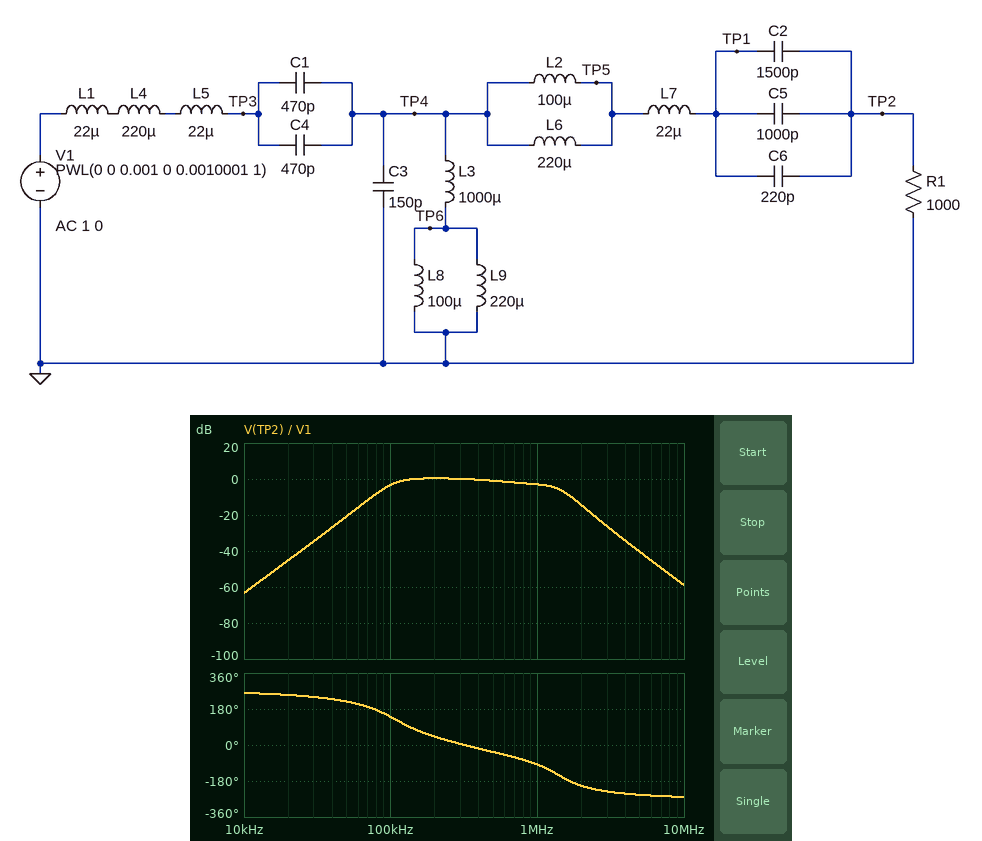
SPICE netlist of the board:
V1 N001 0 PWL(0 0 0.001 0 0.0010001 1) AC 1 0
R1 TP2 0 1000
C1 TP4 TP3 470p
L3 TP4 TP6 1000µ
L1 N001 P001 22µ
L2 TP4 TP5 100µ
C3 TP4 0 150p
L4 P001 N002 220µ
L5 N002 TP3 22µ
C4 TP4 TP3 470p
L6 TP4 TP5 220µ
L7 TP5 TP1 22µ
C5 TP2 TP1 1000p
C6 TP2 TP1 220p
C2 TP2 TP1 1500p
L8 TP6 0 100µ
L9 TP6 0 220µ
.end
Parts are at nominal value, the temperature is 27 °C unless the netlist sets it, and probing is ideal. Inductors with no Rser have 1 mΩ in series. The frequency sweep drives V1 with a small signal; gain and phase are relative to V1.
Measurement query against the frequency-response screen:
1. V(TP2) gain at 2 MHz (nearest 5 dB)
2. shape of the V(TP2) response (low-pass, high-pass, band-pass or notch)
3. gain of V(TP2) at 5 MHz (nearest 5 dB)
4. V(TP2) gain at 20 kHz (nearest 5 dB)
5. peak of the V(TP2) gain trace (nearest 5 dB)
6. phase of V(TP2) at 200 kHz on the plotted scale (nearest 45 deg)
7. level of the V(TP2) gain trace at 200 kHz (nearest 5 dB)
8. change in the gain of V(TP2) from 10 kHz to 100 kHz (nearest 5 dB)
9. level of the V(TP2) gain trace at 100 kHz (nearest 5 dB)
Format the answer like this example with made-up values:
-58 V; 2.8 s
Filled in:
-15 dB; band-pass; -40 dB; -45 dB; 0 dB; 45 deg; 0 dB; 60 dB; -5 dB
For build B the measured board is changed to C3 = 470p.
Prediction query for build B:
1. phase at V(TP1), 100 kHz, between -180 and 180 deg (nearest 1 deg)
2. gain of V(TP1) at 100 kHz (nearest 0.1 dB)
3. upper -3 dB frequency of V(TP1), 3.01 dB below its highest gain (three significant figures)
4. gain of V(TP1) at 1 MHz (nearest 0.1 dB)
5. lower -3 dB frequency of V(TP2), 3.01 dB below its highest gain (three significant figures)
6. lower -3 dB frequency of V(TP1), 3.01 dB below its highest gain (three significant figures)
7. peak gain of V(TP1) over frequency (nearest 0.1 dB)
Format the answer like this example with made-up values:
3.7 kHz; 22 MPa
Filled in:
97 deg; -1.4 dB; 688 kHz; -10.0 dB; 354 kHz; 349 kHz; 3.6 dB
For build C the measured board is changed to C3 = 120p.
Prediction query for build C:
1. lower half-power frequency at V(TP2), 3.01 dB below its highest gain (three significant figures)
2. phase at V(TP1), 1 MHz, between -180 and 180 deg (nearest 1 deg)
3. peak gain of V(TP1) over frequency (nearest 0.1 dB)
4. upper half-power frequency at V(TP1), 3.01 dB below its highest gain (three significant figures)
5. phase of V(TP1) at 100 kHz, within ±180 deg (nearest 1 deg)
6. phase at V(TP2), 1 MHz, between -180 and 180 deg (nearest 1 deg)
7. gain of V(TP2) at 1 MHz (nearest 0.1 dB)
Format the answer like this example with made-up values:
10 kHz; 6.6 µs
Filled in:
106 kHz; -90 deg; 0.9 dB; 622 kHz; 111 deg; -86 deg; -3.8 dB
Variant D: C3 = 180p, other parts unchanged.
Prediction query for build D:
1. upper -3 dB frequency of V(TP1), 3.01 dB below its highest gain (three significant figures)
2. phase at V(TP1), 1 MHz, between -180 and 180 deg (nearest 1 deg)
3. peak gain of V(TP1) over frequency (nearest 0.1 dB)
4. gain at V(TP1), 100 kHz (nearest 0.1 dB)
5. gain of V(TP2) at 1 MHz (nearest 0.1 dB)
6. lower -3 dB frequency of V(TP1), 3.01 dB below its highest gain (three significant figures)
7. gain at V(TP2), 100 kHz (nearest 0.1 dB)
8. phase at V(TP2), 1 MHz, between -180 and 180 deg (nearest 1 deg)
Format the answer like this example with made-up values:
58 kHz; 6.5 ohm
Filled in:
981 kHz; -114 deg; 0.6 dB; -2.0 dB; -2.5 dB; 97.3 kHz; -3.2 dB; -110 deg
